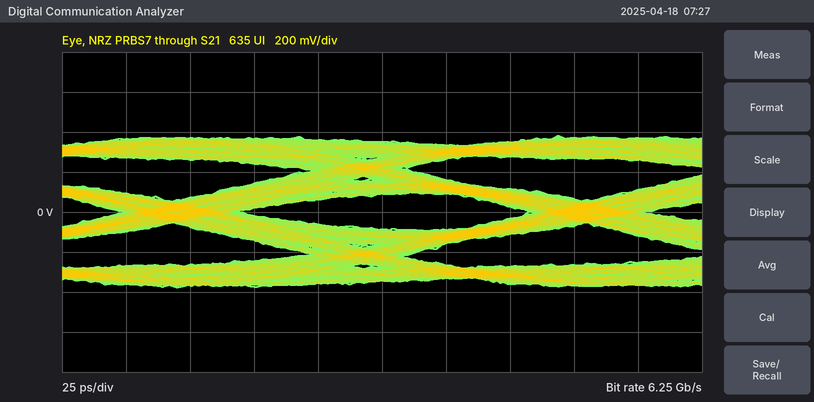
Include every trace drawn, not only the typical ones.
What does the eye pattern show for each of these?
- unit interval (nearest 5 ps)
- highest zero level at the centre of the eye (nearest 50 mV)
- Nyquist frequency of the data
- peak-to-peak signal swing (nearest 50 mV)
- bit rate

160 ps
-100 mV
3.125 GHz
750 mV
6.25 Gb/s
